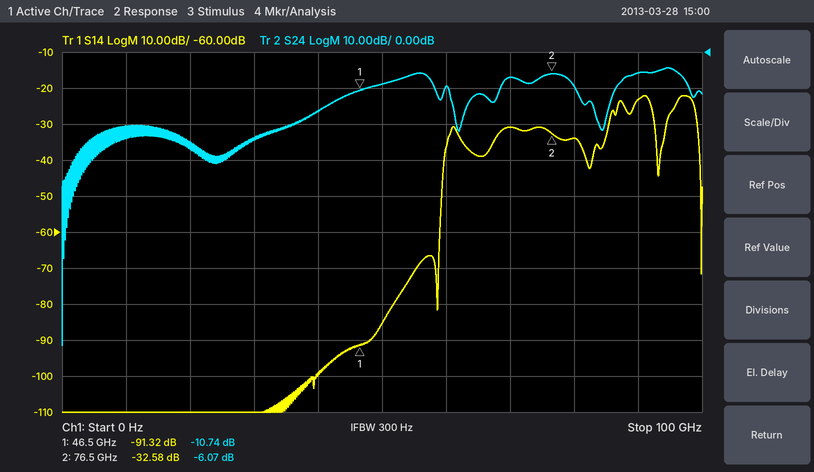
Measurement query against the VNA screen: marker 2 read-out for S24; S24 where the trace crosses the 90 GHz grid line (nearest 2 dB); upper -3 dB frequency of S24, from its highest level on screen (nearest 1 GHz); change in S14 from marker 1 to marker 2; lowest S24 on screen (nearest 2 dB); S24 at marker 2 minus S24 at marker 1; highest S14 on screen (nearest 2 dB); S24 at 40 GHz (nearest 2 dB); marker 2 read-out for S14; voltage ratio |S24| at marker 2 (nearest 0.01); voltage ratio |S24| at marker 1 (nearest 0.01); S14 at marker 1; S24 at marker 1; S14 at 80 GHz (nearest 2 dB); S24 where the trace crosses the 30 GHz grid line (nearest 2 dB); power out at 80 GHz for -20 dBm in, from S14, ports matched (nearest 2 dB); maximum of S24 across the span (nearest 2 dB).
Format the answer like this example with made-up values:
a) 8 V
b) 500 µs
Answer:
a) -6.07 dB
b) -6 dB
c) 97 GHz
d) 58.74 dB
e) -82 dB
f) 4.67 dB
g) -22 dB
h) -16 dB
i) -32.58 dB
j) 0.50
k) 0.29
l) -91.32 dB
m) -10.74 dB
n) -34 dB
o) -24 dB
p) -54 dBm
q) -4 dB
